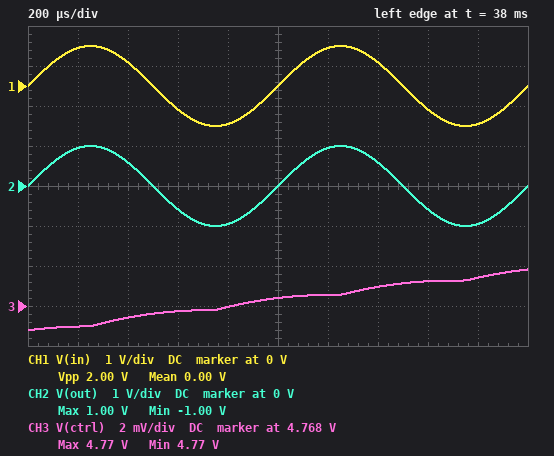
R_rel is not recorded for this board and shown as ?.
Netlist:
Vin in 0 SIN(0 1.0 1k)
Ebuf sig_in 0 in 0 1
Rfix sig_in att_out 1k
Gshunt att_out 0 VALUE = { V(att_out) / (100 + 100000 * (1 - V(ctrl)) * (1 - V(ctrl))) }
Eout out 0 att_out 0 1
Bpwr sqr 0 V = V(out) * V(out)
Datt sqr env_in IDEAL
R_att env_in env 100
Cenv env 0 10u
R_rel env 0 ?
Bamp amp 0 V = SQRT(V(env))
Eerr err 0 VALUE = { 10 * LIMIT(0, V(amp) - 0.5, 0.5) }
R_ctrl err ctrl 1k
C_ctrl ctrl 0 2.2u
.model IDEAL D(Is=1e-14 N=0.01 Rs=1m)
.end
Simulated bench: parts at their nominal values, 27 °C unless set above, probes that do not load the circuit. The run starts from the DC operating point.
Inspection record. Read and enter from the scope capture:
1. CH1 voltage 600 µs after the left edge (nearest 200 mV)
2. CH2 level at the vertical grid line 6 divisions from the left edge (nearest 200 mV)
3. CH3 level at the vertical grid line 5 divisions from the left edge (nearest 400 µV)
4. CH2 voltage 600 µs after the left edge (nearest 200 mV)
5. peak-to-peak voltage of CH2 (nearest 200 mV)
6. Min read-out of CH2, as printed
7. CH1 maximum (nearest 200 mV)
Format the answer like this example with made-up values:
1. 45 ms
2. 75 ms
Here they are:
1. -600 mV
2. 1.0 V
3. 4.7684 V
4. -600 mV
5. 2.0 V
6. -1.00 V
7. 1.0 V
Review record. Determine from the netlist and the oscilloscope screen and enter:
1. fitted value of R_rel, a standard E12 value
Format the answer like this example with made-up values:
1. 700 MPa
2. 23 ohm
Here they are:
1. 33 kΩ
